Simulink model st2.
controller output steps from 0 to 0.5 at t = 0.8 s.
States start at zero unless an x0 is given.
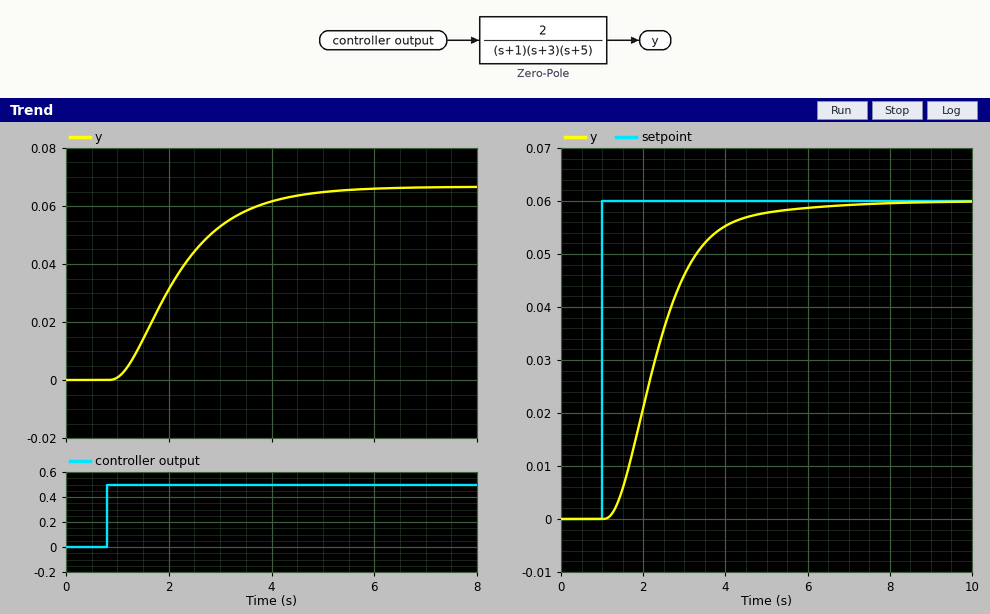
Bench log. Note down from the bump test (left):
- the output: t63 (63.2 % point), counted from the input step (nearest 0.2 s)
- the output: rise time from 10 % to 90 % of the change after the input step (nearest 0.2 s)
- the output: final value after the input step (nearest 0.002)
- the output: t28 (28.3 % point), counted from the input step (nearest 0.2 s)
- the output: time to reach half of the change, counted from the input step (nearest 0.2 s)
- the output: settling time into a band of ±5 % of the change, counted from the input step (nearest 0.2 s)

1.6 s
2.4 s
0.066
0.8 s
1.2 s
3.6 s
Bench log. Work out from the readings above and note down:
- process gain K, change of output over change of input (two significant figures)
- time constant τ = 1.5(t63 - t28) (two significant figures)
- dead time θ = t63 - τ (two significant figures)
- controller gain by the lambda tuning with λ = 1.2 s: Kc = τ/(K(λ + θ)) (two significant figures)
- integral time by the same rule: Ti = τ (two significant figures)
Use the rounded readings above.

0.13
1.2 s
0.40 s
5.8
1.2 s
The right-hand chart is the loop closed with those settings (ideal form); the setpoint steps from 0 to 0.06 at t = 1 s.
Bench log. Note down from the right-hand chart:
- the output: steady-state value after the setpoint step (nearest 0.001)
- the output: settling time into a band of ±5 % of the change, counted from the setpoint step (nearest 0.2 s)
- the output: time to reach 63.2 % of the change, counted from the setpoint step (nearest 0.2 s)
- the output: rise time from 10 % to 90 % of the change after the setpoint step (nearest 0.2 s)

0.060
3.6 s
1.6 s
2.2 s
